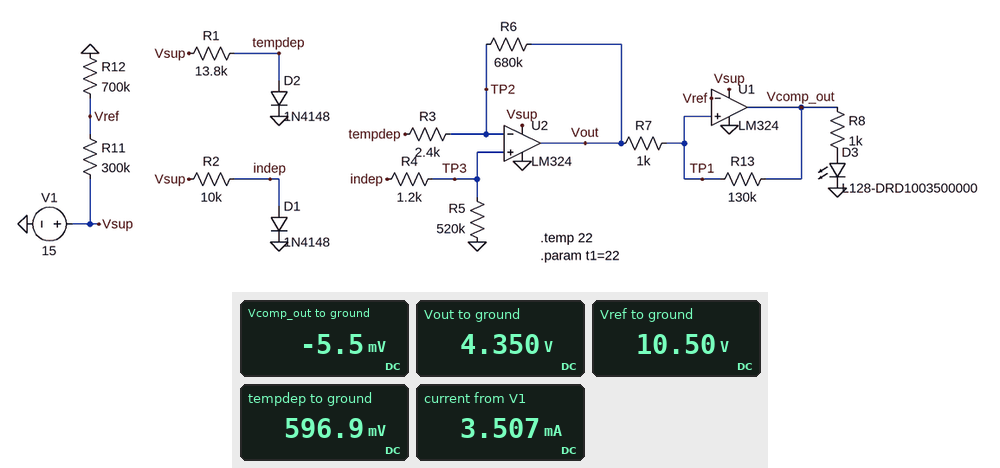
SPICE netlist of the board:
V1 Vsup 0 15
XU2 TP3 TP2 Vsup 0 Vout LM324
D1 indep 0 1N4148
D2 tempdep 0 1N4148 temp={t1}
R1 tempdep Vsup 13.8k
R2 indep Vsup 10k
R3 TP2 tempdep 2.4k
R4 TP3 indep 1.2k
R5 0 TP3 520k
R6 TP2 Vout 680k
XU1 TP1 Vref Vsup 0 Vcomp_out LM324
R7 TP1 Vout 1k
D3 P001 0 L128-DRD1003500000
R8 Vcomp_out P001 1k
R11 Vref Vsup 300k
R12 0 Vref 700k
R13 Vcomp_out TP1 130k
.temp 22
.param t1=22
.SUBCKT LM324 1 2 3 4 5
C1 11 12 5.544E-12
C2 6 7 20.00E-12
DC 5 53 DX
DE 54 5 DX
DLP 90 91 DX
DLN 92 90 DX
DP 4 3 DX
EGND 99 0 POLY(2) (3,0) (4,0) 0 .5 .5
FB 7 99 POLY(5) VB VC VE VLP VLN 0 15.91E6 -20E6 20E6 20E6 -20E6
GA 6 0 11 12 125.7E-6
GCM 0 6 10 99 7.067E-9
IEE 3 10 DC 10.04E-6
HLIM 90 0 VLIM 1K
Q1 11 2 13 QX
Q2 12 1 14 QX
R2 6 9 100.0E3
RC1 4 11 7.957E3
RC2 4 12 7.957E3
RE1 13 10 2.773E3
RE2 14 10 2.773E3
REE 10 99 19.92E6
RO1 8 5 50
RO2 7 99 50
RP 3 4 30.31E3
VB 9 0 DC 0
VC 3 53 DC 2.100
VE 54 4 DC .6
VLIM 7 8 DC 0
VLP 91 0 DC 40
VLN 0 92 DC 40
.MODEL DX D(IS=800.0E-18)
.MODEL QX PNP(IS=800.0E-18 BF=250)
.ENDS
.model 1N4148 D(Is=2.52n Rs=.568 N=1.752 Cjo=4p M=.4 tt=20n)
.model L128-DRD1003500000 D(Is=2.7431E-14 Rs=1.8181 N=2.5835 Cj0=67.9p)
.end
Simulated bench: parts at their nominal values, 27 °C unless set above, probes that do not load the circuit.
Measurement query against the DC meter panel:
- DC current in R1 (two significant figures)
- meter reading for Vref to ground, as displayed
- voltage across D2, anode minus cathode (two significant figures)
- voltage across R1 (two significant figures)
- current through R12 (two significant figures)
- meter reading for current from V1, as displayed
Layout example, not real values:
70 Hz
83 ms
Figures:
1.0 mA
10.50 V
600 mV
14 V
15 µA
3.507 mA
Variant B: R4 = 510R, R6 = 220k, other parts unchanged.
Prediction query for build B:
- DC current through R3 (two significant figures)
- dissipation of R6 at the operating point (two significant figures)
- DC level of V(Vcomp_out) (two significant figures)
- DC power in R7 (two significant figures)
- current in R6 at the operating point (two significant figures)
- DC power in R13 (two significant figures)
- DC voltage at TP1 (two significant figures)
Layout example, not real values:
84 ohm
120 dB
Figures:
5.9 µA
7.5 µW
-5.8 mV
210 nW
5.8 µA
27 µW
1.9 V
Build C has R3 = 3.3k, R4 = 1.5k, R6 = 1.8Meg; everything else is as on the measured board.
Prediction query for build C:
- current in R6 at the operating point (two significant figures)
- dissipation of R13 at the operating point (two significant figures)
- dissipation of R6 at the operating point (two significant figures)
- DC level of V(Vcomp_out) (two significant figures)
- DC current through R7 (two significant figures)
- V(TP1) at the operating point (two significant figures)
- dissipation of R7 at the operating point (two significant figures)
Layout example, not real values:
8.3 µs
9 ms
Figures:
3.9 µA
440 µW
27 µW
-5.2 mV
58 µA
7.6 V
3.4 µW
